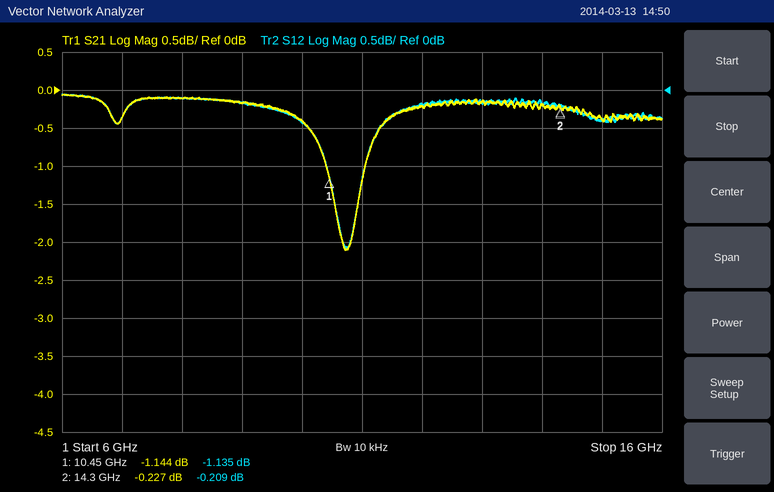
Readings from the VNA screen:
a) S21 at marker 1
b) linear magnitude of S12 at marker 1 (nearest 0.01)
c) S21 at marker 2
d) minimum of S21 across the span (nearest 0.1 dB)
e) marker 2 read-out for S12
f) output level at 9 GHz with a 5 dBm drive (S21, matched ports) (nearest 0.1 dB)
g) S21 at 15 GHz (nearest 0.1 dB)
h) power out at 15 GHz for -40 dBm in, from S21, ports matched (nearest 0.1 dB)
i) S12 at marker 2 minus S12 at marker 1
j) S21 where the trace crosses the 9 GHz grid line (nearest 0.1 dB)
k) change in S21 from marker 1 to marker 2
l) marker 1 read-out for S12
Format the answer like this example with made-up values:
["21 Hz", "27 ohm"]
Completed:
["-1.144 dB", "0.88", "-0.227 dB", "-2.1 dB", "-0.209 dB", "4.8 dBm", "-0.4 dB", "-40.4 dBm", "0.926 dB", "-0.2 dB", "0.917 dB", "-1.135 dB"]
